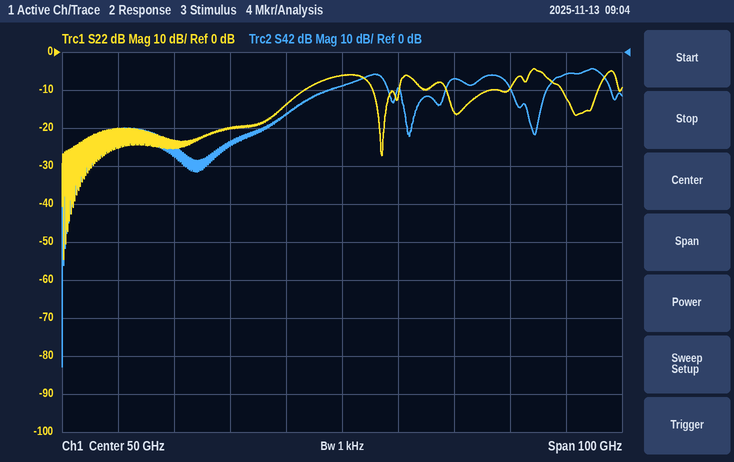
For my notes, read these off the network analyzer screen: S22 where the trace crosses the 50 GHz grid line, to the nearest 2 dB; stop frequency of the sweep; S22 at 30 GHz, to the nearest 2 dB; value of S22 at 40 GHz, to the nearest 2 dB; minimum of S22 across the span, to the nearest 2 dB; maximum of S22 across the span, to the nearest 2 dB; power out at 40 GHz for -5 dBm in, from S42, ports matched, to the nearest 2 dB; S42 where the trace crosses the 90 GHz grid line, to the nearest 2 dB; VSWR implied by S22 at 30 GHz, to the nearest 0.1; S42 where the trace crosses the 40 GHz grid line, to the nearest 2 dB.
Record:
-6 dB
100 GHz
-20 dB
-14 dB
-54 dB
-4 dB
-22 dBm
-6 dB
1.2
-16 dB
